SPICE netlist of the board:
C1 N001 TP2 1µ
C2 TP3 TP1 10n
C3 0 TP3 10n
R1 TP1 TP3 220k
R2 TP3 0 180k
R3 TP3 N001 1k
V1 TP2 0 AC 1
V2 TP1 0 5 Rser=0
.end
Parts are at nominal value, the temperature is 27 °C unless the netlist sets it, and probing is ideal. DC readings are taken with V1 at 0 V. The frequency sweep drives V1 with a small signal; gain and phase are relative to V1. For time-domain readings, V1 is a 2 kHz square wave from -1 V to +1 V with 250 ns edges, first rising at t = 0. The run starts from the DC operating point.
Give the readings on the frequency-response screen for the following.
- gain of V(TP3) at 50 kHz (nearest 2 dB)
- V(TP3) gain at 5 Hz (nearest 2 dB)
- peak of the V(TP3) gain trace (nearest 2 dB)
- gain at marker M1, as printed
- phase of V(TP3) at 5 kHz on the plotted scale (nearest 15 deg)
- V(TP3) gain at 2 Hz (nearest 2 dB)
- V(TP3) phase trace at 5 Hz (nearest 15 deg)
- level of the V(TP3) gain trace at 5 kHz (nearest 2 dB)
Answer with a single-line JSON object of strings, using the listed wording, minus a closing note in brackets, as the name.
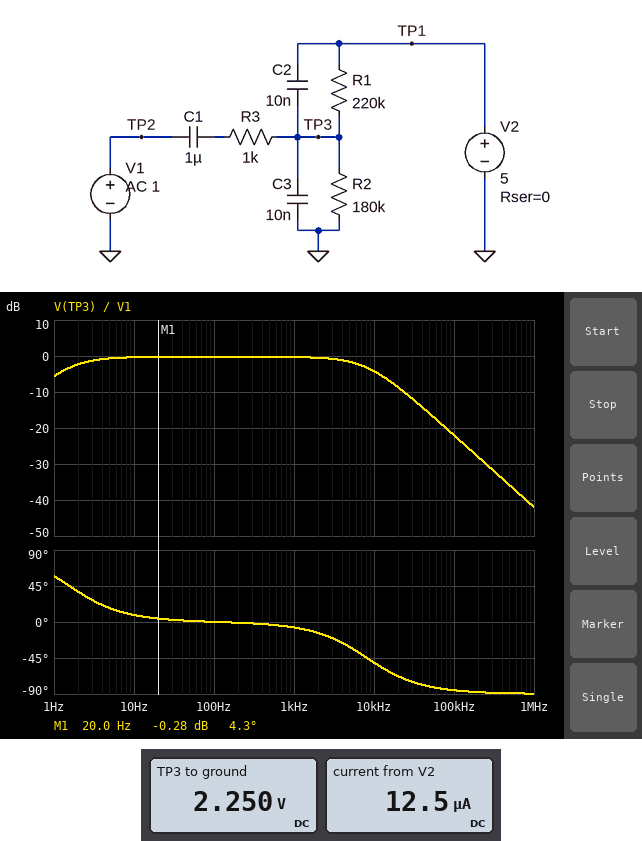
{"gain of V(TP3) at 50 kHz": "-16 dB", "V(TP3) gain at 5 Hz": "0 dB", "peak of the V(TP3) gain trace": "0 dB", "gain at marker M1, as printed": "-0.28 dB", "phase of V(TP3) at 5 kHz on the plotted scale": "-30 deg", "V(TP3) gain at 2 Hz": "-2 dB", "V(TP3) phase trace at 5 Hz": "15 deg", "level of the V(TP3) gain trace at 5 kHz": "-2 dB"}
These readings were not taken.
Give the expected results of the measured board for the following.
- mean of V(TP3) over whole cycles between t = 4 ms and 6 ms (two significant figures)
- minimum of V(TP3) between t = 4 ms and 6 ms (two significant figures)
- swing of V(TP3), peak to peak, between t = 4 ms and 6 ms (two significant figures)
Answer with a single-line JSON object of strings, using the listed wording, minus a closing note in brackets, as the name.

{"mean of V(TP3) over whole cycles between t = 4 ms and 6 ms": "3.2 V", "minimum of V(TP3) between t = 4 ms and 6 ms": "2.2 V", "swing of V(TP3), peak to peak, between t = 4 ms and 6 ms": "2.0 V"}
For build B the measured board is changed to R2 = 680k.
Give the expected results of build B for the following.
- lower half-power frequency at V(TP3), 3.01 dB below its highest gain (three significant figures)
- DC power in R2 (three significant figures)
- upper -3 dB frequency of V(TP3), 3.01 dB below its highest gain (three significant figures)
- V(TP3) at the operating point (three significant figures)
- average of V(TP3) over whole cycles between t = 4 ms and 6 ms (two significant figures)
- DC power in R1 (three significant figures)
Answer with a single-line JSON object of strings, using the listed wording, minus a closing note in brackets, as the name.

{"lower half-power frequency at V(TP3), 3.01 dB below its highest gain": "933 mHz", "DC power in R2": "21.0 µW", "upper -3 dB frequency of V(TP3), 3.01 dB below its highest gain": "8.17 kHz", "V(TP3) at the operating point": "3.78 V", "average of V(TP3) over whole cycles between t = 4 ms and 6 ms": "4.7 V", "DC power in R1": "6.79 µW"}
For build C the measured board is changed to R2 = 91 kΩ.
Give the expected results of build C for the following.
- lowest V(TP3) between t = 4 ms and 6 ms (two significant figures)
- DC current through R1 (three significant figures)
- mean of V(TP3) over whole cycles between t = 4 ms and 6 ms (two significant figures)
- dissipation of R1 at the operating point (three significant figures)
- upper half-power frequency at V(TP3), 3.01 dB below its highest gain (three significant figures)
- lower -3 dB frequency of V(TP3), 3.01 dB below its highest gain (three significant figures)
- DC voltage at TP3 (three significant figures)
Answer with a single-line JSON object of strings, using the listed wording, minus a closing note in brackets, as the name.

{"lowest V(TP3) between t = 4 ms and 6 ms": "1.4 V", "DC current through R1": "16.1 µA", "mean of V(TP3) over whole cycles between t = 4 ms and 6 ms": "2.4 V", "dissipation of R1 at the operating point": "56.9 µW", "upper half-power frequency at V(TP3), 3.01 dB below its highest gain": "8.24 kHz", "lower -3 dB frequency of V(TP3), 3.01 dB below its highest gain": "2.39 Hz", "DC voltage at TP3": "1.46 V"}
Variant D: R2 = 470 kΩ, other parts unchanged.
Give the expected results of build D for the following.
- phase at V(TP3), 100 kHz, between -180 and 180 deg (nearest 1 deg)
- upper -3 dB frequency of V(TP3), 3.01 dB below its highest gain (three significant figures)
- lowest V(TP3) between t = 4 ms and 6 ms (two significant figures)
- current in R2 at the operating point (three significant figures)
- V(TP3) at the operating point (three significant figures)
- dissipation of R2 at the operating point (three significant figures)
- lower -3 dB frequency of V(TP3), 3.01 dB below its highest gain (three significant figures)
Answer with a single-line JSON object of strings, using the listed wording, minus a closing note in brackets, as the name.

{"phase at V(TP3), 100 kHz, between -180 and 180 deg": "-85 deg", "upper -3 dB frequency of V(TP3), 3.01 dB below its highest gain": "8.17 kHz", "lowest V(TP3) between t = 4 ms and 6 ms": "3.4 V", "current in R2 at the operating point": "7.25 µA", "V(TP3) at the operating point": "3.41 V", "dissipation of R2 at the operating point": "24.7 µW", "lower -3 dB frequency of V(TP3), 3.01 dB below its highest gain": "1.03 Hz"}
